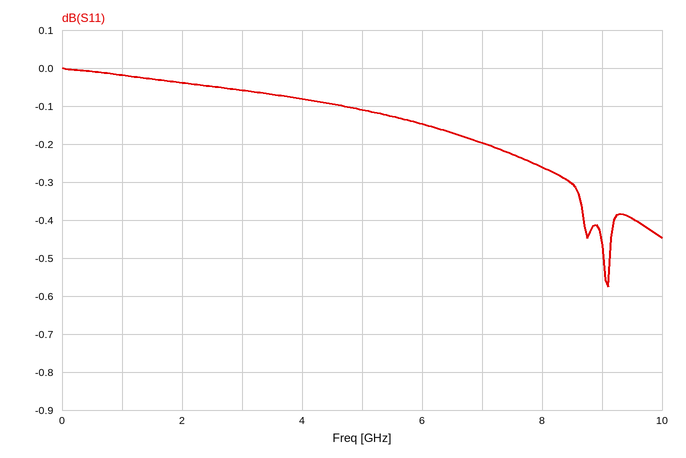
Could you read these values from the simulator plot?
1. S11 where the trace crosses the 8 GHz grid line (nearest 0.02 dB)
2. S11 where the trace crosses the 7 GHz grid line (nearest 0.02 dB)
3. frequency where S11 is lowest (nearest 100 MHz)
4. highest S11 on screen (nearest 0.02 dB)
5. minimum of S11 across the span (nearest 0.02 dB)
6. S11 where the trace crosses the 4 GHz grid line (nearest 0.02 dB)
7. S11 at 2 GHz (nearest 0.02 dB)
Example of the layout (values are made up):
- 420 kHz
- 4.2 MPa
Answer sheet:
- -0.26 dB
- -0.20 dB
- 9.1 GHz
- 0.00 dB
- -0.58 dB
- -0.08 dB
- -0.04 dB
